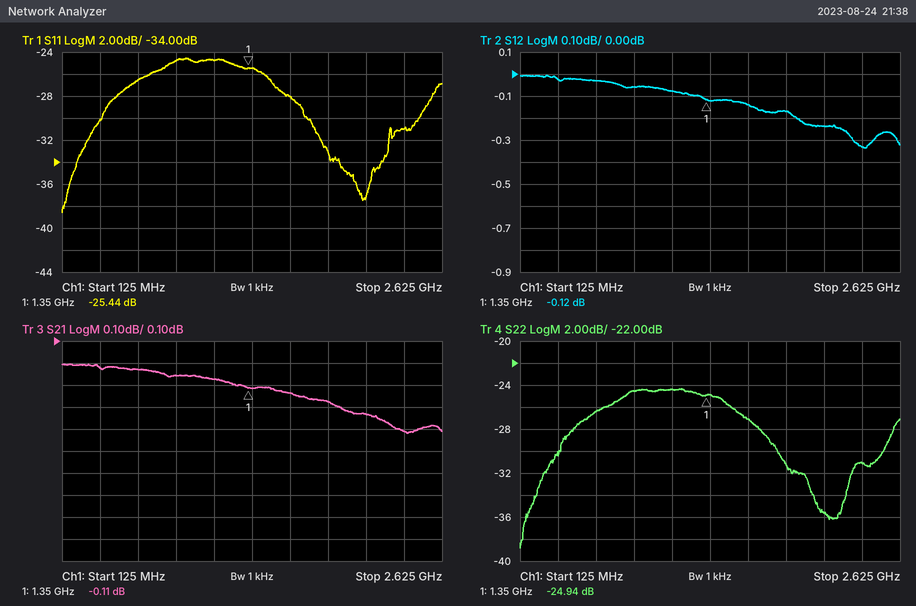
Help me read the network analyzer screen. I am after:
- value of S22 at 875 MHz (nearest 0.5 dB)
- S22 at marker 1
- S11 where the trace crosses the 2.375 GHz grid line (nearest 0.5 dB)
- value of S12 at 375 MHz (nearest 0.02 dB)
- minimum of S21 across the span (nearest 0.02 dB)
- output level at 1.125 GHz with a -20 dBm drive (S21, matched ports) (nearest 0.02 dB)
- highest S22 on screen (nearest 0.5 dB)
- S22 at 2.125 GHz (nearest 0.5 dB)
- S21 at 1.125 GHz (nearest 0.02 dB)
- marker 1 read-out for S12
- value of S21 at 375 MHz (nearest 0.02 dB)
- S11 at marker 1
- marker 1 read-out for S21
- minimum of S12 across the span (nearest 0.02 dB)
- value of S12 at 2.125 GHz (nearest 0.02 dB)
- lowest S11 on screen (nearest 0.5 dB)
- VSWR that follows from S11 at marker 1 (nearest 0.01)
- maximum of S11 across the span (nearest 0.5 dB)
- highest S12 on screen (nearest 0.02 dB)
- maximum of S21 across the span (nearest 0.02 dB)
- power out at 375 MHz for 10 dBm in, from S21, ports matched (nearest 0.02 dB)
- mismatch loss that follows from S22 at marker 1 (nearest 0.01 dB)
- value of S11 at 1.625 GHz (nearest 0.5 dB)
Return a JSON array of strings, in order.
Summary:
["-24.5 dB", "-24.94 dB", "-31.0 dB", "-0.02 dB", "-0.32 dB", "-20.08 dBm", "-24.5 dB", "-35.5 dB", "-0.08 dB", "-0.12 dB", "-0.02 dB", "-25.44 dB", "-0.11 dB", "-0.34 dB", "-0.24 dB", "-38.5 dB", "1.11", "-24.5 dB", "0.00 dB", "0.00 dB", "9.98 dBm", "0.01 dB", "-28.0 dB"]
